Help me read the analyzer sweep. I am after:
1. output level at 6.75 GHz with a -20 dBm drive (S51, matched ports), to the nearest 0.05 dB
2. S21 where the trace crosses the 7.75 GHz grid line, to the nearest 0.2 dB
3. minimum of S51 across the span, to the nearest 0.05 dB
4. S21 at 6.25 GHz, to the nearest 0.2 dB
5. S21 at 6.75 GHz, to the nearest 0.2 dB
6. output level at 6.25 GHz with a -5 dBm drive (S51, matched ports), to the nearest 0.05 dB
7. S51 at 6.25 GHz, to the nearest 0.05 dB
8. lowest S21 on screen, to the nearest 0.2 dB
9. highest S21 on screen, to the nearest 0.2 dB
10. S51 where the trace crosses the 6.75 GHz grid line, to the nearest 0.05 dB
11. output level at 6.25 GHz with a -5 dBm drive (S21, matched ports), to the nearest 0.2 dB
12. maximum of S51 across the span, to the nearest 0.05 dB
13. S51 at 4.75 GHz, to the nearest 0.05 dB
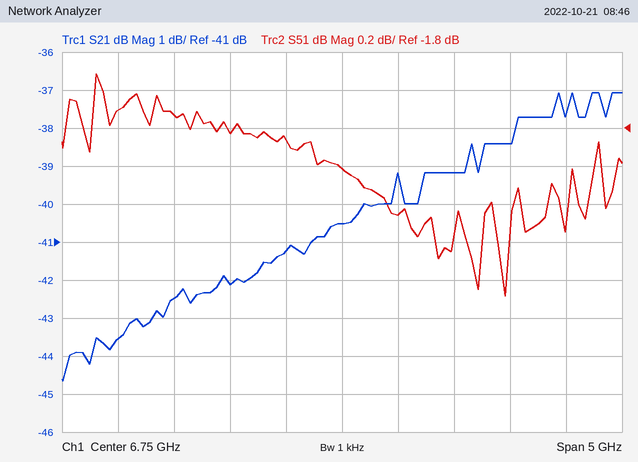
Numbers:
-22.00 dBm
-39.2 dB
-2.70 dB
-41.2 dB
-40.6 dB
-6.85 dBm
-1.85 dB
-44.6 dB
-37.0 dB
-2.00 dB
-46.2 dBm
-1.50 dB
-1.70 dB
